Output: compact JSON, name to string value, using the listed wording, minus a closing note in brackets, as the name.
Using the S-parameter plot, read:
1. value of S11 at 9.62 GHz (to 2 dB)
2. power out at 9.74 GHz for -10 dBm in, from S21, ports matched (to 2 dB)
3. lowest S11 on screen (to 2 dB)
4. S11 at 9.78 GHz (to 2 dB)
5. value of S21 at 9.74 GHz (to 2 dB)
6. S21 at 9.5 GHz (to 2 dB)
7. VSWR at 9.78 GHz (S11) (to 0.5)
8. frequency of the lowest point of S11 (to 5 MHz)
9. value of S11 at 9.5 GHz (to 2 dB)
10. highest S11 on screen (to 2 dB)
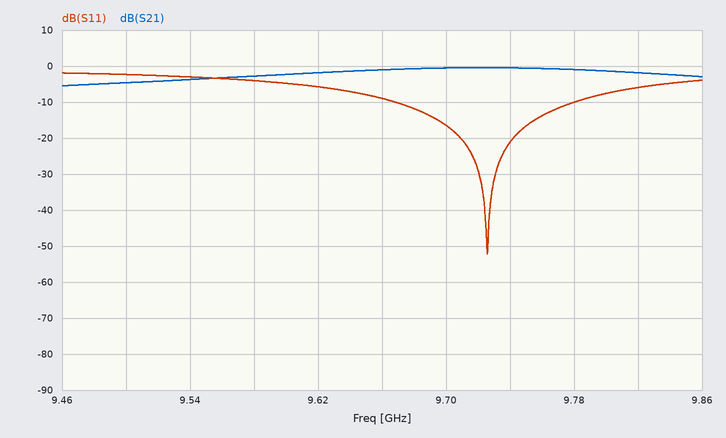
{"value of S11 at 9.62 GHz": "-6 dB", "power out at 9.74 GHz for -10 dBm in, from S21, ports matched": "-10 dBm", "lowest S11 on screen": "-52 dB", "S11 at 9.78 GHz": "-10 dB", "value of S21 at 9.74 GHz": "0 dB", "S21 at 9.5 GHz": "-4 dB", "VSWR at 9.78 GHz (S11)": "2.0", "frequency of the lowest point of S11": "9.725 GHz", "value of S11 at 9.5 GHz": "-2 dB", "highest S11 on screen": "-2 dB"}
